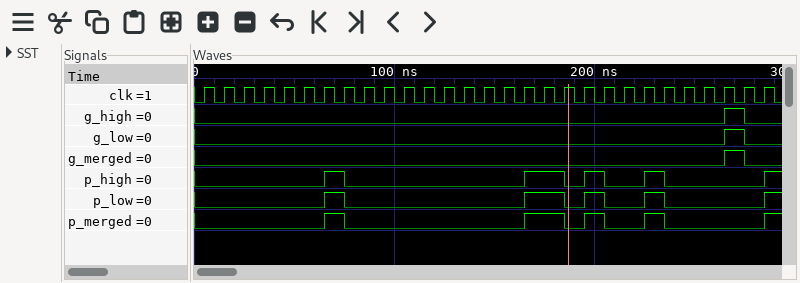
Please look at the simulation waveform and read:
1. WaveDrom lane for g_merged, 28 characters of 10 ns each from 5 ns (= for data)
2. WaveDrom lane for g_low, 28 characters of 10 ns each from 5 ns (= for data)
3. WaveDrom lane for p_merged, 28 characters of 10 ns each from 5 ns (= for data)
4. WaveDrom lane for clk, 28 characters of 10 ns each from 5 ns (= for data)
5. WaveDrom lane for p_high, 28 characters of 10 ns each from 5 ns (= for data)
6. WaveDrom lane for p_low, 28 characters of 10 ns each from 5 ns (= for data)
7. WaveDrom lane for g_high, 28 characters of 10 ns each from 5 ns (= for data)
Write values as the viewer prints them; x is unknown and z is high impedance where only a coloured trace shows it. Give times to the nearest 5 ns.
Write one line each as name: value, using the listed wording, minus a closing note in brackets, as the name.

WaveDrom lane for g_merged, 28 characters of 10 ns each from 5 ns: {name: 'g_merged', wave: '0.........................10'}
WaveDrom lane for g_low, 28 characters of 10 ns each from 5 ns: {name: 'g_low', wave: '0.........................10'}
WaveDrom lane for p_merged, 28 characters of 10 ns each from 5 ns: {name: 'p_merged', wave: '0.....10........1.010.10....'}
WaveDrom lane for clk, 28 characters of 10 ns each from 5 ns: {name: 'clk', wave: 'p...........................'}
WaveDrom lane for p_high, 28 characters of 10 ns each from 5 ns: {name: 'p_high', wave: '0.....10........1.010.10....'}
WaveDrom lane for p_low, 28 characters of 10 ns each from 5 ns: {name: 'p_low', wave: '0.....10........1.010.10....'}
WaveDrom lane for g_high, 28 characters of 10 ns each from 5 ns: {name: 'g_high', wave: '0.........................10'}
